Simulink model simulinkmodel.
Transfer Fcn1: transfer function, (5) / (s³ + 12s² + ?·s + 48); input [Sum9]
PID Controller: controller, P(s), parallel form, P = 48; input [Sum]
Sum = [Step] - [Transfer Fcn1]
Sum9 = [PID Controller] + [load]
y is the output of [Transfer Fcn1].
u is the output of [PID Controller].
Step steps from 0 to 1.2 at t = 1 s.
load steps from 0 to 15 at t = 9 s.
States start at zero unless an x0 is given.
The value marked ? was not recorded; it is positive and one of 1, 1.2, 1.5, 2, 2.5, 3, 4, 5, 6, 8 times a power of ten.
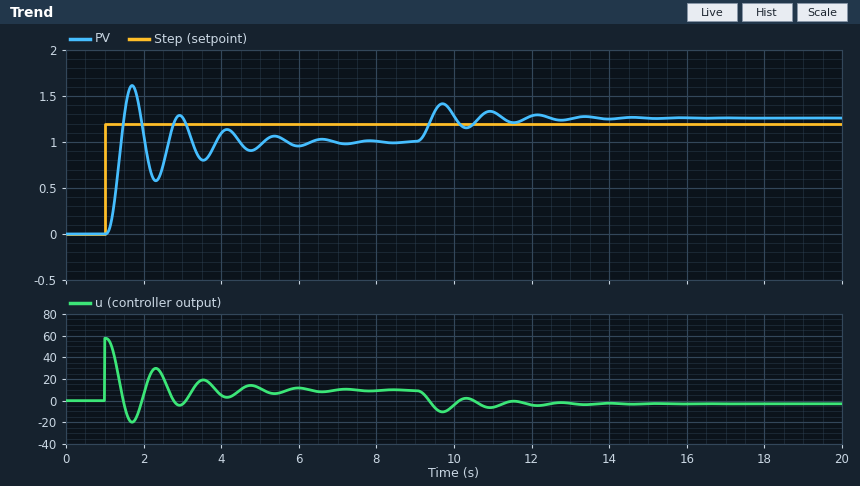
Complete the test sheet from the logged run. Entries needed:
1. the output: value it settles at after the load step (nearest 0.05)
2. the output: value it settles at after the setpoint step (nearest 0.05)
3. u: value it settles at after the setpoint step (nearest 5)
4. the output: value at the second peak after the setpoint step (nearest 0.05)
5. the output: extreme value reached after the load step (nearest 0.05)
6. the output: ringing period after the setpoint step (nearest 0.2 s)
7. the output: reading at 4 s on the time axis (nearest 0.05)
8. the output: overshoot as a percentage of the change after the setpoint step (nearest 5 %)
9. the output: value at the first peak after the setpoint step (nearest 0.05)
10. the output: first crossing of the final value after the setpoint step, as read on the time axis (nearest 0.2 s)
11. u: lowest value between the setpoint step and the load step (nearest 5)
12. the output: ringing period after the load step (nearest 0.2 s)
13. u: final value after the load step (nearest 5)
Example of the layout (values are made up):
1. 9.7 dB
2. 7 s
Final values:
1. 1.25
2. 1.00
3. 10
4. 1.30
5. 1.40
6. 1.2 s
7. 1.10
8. 60 %
9. 1.60
10. 1.4 s
11. -20
12. 1.2 s
13. -5
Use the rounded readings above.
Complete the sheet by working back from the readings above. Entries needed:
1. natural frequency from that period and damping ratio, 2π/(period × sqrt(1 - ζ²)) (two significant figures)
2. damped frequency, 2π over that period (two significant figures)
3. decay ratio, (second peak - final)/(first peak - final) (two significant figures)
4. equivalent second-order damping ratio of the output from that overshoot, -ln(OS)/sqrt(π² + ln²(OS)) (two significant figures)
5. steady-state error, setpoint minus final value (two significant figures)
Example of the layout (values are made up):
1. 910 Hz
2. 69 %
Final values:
1. 5.3 rad/s
2. 5.2 rad/s
3. 0.50
4. 0.16
5. 0.20
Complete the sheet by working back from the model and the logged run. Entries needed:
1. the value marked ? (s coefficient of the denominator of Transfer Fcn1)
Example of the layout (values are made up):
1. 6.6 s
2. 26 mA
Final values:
1. 40
